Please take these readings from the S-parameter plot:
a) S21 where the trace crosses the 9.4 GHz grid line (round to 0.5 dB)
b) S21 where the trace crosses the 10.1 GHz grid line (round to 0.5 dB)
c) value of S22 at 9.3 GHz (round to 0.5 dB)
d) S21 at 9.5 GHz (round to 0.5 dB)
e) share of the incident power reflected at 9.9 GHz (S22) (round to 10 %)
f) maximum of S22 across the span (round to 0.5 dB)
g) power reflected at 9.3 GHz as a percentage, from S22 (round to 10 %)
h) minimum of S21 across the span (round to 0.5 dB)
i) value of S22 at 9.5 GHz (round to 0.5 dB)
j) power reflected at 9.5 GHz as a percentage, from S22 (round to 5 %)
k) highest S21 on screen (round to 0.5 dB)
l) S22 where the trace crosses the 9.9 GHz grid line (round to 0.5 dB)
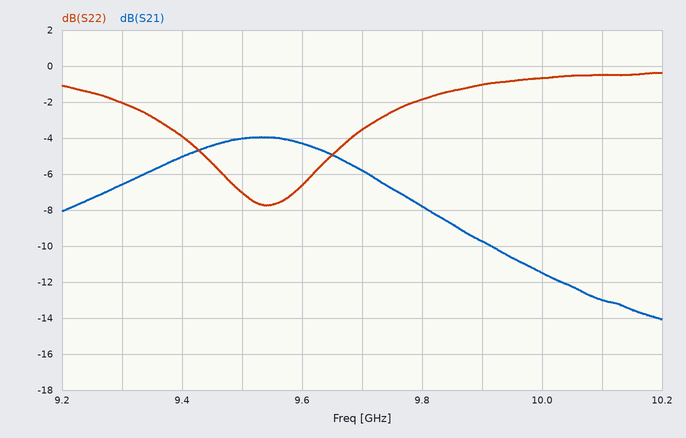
-5.0 dB
-13.0 dB
-2.0 dB
-4.0 dB
80 %
-0.5 dB
60 %
-14.0 dB
-7.0 dB
20 %
-4.0 dB
-1.0 dB
